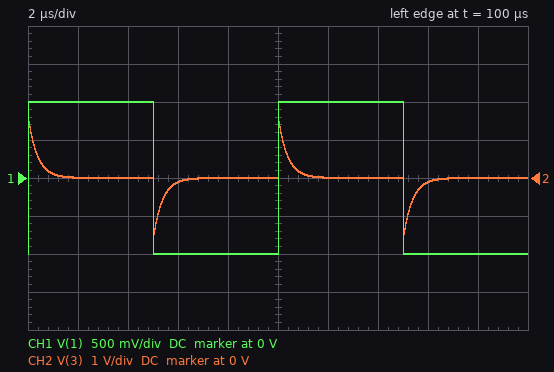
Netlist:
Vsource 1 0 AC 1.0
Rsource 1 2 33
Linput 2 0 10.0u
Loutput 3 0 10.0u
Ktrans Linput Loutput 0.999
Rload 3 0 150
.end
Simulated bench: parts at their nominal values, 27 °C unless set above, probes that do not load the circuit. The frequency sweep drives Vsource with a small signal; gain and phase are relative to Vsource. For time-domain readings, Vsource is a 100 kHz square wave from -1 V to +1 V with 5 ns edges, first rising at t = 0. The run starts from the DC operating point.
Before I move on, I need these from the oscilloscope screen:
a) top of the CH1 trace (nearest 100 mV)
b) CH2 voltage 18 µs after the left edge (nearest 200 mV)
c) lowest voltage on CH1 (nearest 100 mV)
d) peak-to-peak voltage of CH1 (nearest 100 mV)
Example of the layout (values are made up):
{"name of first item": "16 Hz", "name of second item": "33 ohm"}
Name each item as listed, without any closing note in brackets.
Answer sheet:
{"top of the CH1 trace": "1.0 V", "CH2 voltage 18 µs after the left edge": "0 V", "lowest voltage on CH1": "-1.0 V", "peak-to-peak voltage of CH1": "2.0 V"}
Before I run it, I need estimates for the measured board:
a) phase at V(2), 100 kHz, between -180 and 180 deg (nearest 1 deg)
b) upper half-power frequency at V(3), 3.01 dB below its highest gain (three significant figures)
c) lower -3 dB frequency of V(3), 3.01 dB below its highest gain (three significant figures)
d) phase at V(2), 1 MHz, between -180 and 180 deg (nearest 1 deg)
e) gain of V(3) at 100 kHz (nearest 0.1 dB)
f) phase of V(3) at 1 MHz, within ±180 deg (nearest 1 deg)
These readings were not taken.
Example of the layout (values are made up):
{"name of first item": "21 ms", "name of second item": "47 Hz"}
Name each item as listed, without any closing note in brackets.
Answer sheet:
{"phase at V(2), 100 kHz, between -180 and 180 deg": "77 deg", "upper half-power frequency at V(3), 3.01 dB below its highest gain": "1.46 GHz", "lower -3 dB frequency of V(3), 3.01 dB below its highest gain": "430 kHz", "phase at V(2), 1 MHz, between -180 and 180 deg": "23 deg", "gain of V(3) at 100 kHz": "-14.6 dB", "phase of V(3) at 1 MHz, within ±180 deg": "23 deg"}
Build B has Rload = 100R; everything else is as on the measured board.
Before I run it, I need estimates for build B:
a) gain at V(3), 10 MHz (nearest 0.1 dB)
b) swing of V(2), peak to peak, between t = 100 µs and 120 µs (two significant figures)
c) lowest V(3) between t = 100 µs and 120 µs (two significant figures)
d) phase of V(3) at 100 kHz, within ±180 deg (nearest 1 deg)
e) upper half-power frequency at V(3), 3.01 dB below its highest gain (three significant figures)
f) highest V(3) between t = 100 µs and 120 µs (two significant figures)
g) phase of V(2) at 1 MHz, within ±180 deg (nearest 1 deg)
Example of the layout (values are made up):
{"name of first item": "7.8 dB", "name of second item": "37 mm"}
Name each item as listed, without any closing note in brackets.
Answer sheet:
{"gain at V(3), 10 MHz": "-2.5 dB", "swing of V(2), peak to peak, between t = 100 µs and 120 µs": "3.0 V", "lowest V(3) between t = 100 µs and 120 µs": "-1.5 V", "phase of V(3) at 100 kHz, within ±180 deg": "76 deg", "upper half-power frequency at V(3), 3.01 dB below its highest gain": "1.06 GHz", "highest V(3) between t = 100 µs and 120 µs": "1.5 V", "phase of V(2) at 1 MHz, within ±180 deg": "22 deg"}
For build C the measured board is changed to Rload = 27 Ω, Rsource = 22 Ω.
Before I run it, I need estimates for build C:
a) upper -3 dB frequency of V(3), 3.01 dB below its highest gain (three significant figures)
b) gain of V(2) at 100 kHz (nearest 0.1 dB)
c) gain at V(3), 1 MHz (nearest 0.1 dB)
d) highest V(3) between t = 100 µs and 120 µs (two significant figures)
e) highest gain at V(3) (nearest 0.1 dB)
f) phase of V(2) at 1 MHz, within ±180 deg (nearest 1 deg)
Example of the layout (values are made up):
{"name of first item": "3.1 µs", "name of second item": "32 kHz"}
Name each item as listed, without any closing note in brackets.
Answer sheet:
{"upper -3 dB frequency of V(3), 3.01 dB below its highest gain": "390 MHz", "gain of V(2) at 100 kHz": "-11.9 dB", "gain at V(3), 1 MHz": "-5.3 dB", "highest V(3) between t = 100 µs and 120 µs": "1.1 V", "highest gain at V(3)": "-5.2 dB", "phase of V(2) at 1 MHz, within ±180 deg": "11 deg"}
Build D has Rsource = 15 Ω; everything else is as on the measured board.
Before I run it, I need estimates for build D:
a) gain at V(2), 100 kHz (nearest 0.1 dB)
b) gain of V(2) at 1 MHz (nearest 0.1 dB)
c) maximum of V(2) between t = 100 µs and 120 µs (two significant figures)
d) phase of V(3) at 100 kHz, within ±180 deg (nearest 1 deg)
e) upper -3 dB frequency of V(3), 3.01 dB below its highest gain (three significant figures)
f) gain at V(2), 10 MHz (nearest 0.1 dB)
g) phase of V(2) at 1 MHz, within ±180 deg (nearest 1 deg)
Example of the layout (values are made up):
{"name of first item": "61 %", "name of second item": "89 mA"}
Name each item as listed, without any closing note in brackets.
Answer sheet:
{"gain at V(2), 100 kHz": "-8.4 dB", "gain of V(2) at 1 MHz": "-1.0 dB", "maximum of V(2) between t = 100 µs and 120 µs": "1.8 V", "phase of V(3) at 100 kHz, within ±180 deg": "65 deg", "upper -3 dB frequency of V(3), 3.01 dB below its highest gain": "1.31 GHz", "gain at V(2), 10 MHz": "-0.8 dB", "phase of V(2) at 1 MHz, within ±180 deg": "12 deg"}
